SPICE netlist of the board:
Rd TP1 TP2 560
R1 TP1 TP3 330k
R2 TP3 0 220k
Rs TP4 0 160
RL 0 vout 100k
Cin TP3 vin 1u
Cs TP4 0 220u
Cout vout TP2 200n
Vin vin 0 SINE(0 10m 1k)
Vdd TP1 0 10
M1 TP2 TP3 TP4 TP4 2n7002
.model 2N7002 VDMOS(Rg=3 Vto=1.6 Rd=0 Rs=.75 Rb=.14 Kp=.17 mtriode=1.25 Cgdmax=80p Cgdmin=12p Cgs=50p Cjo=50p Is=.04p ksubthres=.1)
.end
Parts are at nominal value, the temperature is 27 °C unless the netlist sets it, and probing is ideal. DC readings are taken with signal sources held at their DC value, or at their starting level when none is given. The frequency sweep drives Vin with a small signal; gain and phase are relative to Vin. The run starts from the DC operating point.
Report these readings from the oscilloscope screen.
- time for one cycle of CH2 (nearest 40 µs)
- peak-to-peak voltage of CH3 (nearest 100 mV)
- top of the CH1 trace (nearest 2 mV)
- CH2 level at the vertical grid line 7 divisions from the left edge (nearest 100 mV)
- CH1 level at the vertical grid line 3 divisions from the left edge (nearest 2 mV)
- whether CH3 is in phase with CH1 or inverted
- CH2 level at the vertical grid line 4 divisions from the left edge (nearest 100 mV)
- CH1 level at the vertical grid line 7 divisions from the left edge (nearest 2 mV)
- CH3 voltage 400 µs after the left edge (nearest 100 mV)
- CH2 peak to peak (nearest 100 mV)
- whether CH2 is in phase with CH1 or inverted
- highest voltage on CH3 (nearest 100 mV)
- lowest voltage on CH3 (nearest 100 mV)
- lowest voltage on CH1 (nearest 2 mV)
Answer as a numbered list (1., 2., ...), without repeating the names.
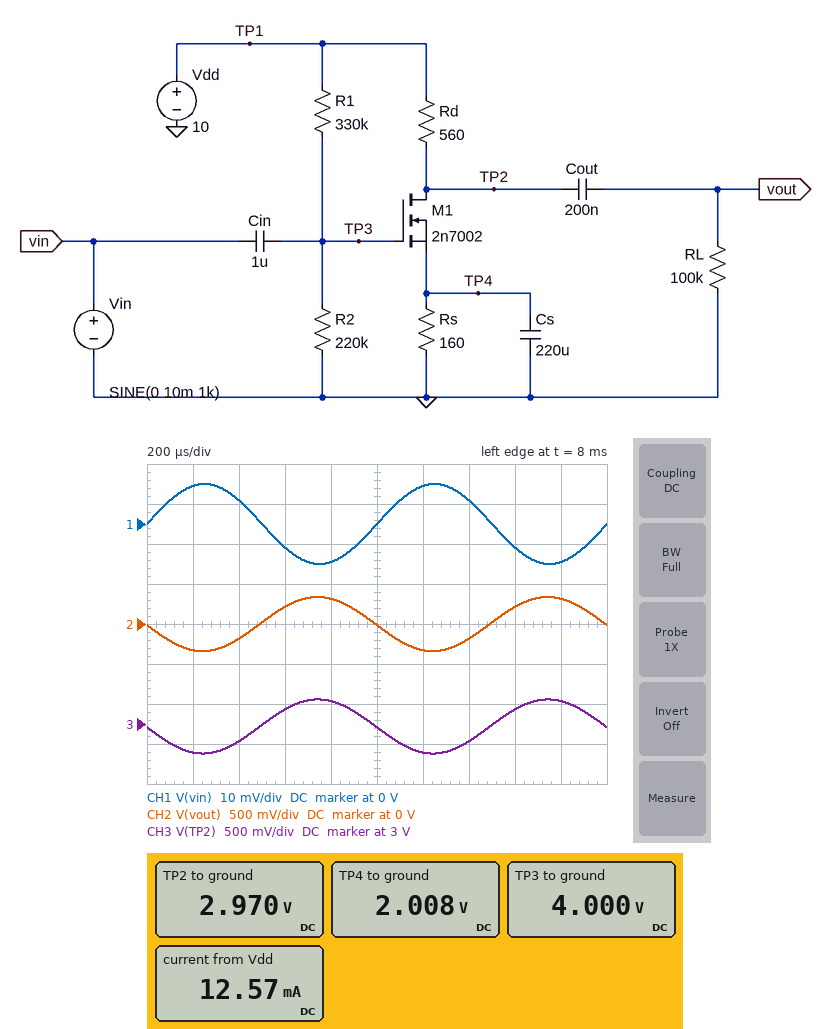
1. 1.00 ms
2. 700 mV
3. 10 mV
4. -200 mV
5. -6 mV
6. inverted
7. 300 mV
8. 6 mV
9. 2.8 V
10. 700 mV
11. inverted
12. 3.3 V
13. 2.6 V
14. -10 mV
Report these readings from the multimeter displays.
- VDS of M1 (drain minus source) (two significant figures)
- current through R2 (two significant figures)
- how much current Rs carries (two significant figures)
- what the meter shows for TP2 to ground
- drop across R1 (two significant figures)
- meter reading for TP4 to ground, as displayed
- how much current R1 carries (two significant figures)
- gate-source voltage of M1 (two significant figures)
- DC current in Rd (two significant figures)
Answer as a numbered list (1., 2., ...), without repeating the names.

1. 960 mV
2. 18 µA
3. 13 mA
4. 2.970 V
5. 6.0 V
6. 2.008 V
7. 18 µA
8. 2.0 V
9. 13 mA
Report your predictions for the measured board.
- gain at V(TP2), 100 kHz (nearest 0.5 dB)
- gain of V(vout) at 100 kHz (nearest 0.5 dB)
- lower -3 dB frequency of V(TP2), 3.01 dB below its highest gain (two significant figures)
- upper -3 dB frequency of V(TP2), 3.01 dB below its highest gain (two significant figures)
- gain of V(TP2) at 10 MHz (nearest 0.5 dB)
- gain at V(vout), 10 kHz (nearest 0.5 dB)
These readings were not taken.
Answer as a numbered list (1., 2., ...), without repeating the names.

1. 30.5 dB
2. 30.5 dB
3. 48 Hz
4. 2.4 MHz
5. 18.0 dB
6. 30.5 dB
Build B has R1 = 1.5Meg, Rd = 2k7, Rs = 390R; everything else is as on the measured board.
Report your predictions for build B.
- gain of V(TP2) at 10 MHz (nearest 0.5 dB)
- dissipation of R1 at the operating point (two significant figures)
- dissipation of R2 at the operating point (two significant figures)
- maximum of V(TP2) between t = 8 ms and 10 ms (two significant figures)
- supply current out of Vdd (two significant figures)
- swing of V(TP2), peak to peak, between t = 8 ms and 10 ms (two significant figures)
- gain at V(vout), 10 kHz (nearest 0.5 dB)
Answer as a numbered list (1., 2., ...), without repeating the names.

1. -6.0 dB
2. 51 µW
3. 7.4 µW
4. 10 V
5. 7.1 µA
6. 1.4 mV
7. -23.5 dB
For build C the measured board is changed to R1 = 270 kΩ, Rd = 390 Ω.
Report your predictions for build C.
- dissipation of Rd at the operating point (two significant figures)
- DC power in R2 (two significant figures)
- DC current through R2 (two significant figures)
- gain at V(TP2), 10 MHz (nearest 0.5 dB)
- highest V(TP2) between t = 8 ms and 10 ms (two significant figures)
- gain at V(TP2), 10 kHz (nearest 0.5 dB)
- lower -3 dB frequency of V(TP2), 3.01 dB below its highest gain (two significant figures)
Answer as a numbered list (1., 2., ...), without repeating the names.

1. 92 mW
2. 92 µW
3. 20 µA
4. 19.5 dB
5. 4.3 V
6. 28.5 dB
7. 53 Hz
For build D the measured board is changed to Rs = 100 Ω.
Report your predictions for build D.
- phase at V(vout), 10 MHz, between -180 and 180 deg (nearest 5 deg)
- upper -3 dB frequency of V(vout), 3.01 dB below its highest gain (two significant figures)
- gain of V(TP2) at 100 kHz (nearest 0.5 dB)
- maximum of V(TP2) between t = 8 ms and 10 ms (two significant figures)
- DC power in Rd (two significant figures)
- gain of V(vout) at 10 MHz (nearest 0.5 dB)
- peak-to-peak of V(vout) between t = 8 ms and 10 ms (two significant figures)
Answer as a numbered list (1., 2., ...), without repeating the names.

1. 155 deg
2. 1.1 GHz
3. -19.5 dB
4. 1.6 V
5. 130 mW
6. -19.0 dB
7. 2.1 mV
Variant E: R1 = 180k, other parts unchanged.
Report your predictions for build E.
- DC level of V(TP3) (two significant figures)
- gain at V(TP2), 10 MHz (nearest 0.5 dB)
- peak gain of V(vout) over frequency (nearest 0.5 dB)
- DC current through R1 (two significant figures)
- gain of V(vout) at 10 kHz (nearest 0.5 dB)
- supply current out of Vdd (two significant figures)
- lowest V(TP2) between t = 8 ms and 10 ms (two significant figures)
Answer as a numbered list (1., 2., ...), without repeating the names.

1. 5.5 V
2. -30.0 dB
3. -8.5 dB
4. 25 µA
5. -32.5 dB
6. 14 mA
7. 2.3 V
